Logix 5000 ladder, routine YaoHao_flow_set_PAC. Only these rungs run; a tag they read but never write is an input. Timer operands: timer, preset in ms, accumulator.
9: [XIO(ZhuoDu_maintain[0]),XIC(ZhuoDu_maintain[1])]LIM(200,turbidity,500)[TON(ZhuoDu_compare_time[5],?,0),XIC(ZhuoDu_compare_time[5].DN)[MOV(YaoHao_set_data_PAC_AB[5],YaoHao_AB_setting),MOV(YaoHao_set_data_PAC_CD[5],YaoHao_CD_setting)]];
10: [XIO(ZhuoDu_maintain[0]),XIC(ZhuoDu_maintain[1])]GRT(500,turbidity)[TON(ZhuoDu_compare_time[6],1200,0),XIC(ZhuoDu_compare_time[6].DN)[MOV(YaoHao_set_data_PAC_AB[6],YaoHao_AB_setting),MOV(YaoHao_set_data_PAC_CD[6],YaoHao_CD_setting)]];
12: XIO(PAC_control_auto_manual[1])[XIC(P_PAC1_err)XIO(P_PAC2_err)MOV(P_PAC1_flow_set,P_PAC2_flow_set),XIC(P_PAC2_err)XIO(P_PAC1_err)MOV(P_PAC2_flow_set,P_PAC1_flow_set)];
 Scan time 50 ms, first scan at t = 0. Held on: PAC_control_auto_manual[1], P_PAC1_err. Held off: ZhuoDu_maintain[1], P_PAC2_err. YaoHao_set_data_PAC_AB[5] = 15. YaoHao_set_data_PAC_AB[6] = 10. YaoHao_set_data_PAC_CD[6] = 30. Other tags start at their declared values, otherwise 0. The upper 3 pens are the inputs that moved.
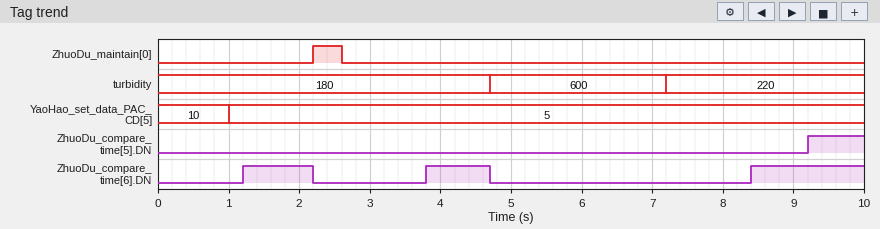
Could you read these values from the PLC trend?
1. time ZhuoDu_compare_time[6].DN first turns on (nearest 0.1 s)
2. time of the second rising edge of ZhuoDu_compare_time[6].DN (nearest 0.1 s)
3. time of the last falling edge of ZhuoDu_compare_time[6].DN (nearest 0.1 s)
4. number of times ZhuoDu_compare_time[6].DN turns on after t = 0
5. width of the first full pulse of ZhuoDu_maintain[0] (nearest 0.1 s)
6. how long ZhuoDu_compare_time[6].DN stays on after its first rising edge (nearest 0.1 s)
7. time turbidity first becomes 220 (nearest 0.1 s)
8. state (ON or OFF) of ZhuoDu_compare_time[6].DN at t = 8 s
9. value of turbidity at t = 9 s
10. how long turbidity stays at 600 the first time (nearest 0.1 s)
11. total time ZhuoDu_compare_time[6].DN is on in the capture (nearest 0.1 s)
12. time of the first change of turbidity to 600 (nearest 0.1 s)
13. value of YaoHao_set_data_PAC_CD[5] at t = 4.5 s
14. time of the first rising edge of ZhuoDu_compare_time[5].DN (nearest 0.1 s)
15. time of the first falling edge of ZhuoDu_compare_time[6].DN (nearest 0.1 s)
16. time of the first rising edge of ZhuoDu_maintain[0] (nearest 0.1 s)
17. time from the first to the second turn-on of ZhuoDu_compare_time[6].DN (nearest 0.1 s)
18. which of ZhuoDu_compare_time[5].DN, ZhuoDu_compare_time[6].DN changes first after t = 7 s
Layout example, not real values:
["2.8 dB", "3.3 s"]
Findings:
["1.2 s", "3.8 s", "4.7 s", "3", "0.4 s", "1.0 s", "7.2 s", "OFF", "220", "2.5 s", "3.5 s", "4.7 s", "5", "9.2 s", "2.2 s", "2.2 s", "2.6 s", "ZhuoDu_compare_time[6].DN"]
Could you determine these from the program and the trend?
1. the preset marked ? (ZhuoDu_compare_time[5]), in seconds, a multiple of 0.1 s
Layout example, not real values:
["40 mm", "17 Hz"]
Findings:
["2.0 s"]
